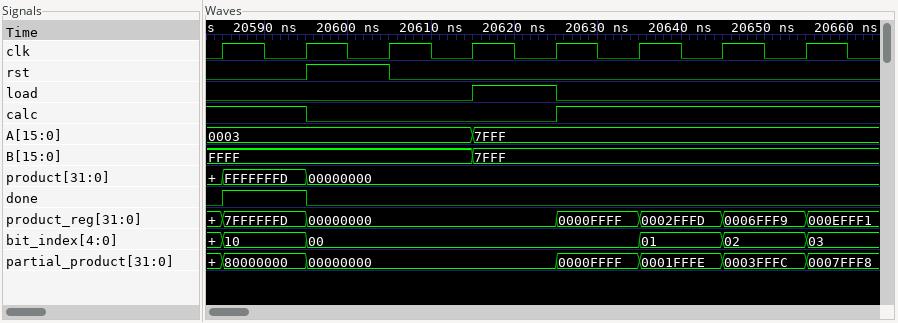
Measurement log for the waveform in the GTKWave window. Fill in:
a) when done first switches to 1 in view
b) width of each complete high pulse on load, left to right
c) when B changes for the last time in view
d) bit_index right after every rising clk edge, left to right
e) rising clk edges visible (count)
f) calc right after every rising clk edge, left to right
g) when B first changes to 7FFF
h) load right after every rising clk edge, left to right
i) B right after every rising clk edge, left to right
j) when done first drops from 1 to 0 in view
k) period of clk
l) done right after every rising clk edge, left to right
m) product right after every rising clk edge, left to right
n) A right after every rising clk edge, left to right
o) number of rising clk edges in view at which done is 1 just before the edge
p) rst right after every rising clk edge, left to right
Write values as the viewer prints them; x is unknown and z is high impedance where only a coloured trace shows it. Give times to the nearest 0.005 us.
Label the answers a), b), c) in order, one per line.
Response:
a) 20.585 us
b) 0.01 us
c) 20.615 us
d) 10, 00, 00, 00, 00, 01, 02, 03
e) 8
f) 1 0 0 0 1 1 1 1
g) 20.615 us
h) 0 0 0 1 0 0 0 0
i) FFFF, FFFF, FFFF, 7FFF, 7FFF, 7FFF, 7FFF, 7FFF
j) 20.595 us
k) 0.01 us
l) 1 0 0 0 0 0 0 0
m) FFFFFFFD, 00000000, 00000000, 00000000, 00000000, 00000000, 00000000, 00000000
n) 0003, 0003, 0003, 7FFF, 7FFF, 7FFF, 7FFF, 7FFF
o) 1
p) 0 1 0 0 0 0 0 0
